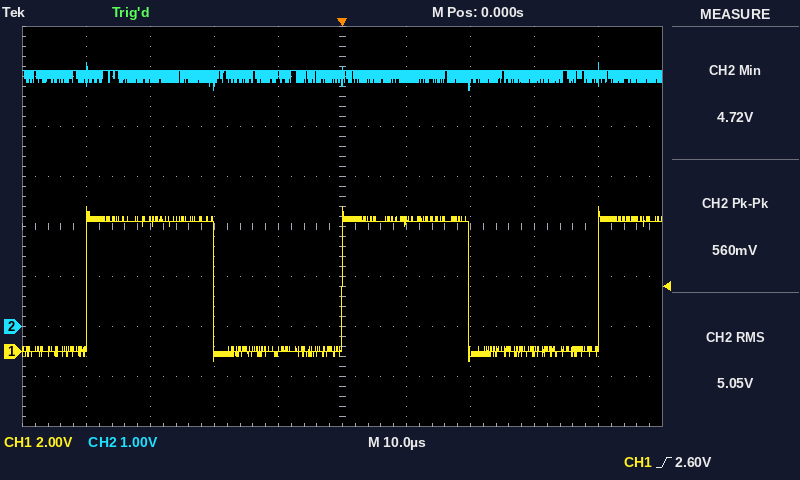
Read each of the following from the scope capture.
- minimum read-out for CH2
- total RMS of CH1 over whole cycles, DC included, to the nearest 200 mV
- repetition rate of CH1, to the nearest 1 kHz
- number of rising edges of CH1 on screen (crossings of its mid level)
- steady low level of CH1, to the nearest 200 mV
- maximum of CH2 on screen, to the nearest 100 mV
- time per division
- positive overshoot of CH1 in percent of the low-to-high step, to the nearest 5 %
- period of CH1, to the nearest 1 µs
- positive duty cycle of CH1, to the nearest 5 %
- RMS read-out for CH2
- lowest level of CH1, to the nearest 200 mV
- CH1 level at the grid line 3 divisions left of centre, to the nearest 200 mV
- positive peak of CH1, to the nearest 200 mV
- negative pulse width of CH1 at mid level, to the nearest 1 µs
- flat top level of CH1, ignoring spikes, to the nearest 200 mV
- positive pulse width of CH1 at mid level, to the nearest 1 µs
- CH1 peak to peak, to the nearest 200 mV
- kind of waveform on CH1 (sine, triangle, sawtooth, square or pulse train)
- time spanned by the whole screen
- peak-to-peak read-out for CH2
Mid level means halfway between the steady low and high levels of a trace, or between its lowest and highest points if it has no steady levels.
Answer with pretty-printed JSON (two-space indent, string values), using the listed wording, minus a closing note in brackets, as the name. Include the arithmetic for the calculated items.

{
  "minimum read-out for CH2": "4.72 V",
  "total RMS of CH1 over whole cycles, DC included, to the nearest 200 mV": "√(0.5 × (5.2 V)² + 0.5 × (0.0 V)²) ≈ 3.68 V, so 3.6 V to the nearest 200 mV",
  "repetition rate of CH1, to the nearest 1 kHz": "1 / 40 µs ≈ 25 kHz",
  "number of rising edges of CH1 on screen": "3",
  "steady low level of CH1, to the nearest 200 mV": "0.0 V",
  "maximum of CH2 on screen, to the nearest 100 mV": "5.3 V",
  "time per division": "10 µs",
  "positive overshoot of CH1 in percent of the low-to-high step, to the nearest 5 %": "10 %",
  "period of CH1, to the nearest 1 µs": "40 µs",
  "positive duty cycle of CH1, to the nearest 5 %": "20 µs / 40 µs ≈ 50 %",
  "RMS read-out for CH2": "5.05 V",
  "lowest level of CH1, to the nearest 200 mV": "-400 mV",
  "CH1 level at the grid line 3 divisions left of centre, to the nearest 200 mV": "5.2 V",
  "positive peak of CH1, to the nearest 200 mV": "5.8 V",
  "negative pulse width of CH1 at mid level, to the nearest 1 µs": "20 µs",
  "flat top level of CH1, ignoring spikes, to the nearest 200 mV": "5.2 V",
  "positive pulse width of CH1 at mid level, to the nearest 1 µs": "20 µs",
  "CH1 peak to peak, to the nearest 200 mV": "5.8 V − (-400 mV) = 6.2 V",
  "kind of waveform on CH1": "square",
  "time spanned by the whole screen": "100 µs",
  "peak-to-peak read-out for CH2": "560 mV"
}
